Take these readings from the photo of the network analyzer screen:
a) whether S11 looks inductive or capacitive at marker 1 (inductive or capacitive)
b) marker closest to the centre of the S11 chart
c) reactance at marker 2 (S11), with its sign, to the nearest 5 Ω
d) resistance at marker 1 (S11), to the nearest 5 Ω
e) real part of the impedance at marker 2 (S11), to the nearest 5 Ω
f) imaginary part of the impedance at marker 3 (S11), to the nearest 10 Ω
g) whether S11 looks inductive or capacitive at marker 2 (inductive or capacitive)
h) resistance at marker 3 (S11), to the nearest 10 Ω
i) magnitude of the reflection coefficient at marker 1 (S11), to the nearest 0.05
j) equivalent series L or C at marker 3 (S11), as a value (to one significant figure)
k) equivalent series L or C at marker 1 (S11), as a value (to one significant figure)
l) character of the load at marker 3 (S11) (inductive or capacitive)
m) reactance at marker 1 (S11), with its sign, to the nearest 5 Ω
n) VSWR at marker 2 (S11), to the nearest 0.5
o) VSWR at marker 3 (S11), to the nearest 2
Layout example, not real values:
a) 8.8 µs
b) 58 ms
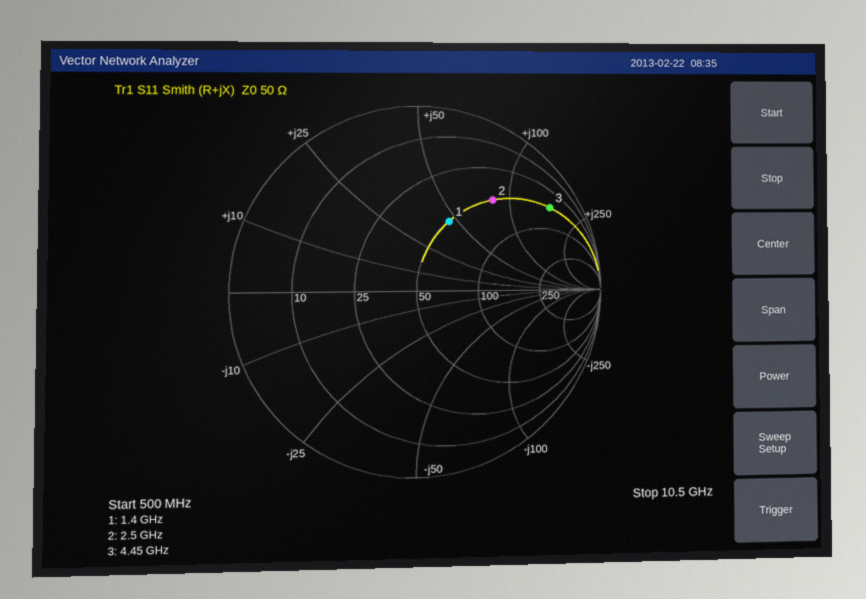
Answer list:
a) inductive
b) marker 1
c) +85 Ω
d) 50 Ω
e) 50 Ω
f) +160 Ω
g) inductive
h) 50 Ω
i) 0.40
j) 6 nH
k) 5 nH
l) inductive
m) +45 Ω
n) 4.5
o) 12
